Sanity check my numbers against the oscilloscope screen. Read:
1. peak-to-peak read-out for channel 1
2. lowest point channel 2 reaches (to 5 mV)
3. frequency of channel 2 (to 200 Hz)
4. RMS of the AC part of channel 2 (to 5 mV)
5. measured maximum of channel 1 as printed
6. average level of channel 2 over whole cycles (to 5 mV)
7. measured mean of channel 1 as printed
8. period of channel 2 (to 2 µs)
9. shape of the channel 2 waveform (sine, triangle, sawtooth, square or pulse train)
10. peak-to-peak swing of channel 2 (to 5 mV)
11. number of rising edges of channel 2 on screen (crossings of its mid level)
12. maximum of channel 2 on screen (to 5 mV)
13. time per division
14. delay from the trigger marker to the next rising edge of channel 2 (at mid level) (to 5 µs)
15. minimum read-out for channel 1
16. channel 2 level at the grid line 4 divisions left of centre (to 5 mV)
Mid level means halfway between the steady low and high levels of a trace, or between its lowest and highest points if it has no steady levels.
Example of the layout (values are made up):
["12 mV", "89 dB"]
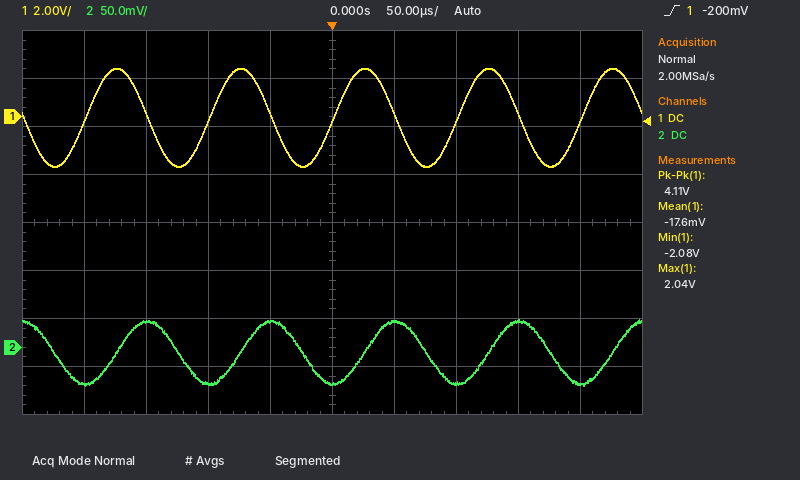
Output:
["4.11 V", "-40 mV", "10.0 kHz", "25 mV", "2.04 V", "-5 mV", "-17.6 mV", "100 µs", "sine", "70 mV", "5", "30 mV", "50 µs", "25 µs", "-2.08 V", "-40 mV"]
